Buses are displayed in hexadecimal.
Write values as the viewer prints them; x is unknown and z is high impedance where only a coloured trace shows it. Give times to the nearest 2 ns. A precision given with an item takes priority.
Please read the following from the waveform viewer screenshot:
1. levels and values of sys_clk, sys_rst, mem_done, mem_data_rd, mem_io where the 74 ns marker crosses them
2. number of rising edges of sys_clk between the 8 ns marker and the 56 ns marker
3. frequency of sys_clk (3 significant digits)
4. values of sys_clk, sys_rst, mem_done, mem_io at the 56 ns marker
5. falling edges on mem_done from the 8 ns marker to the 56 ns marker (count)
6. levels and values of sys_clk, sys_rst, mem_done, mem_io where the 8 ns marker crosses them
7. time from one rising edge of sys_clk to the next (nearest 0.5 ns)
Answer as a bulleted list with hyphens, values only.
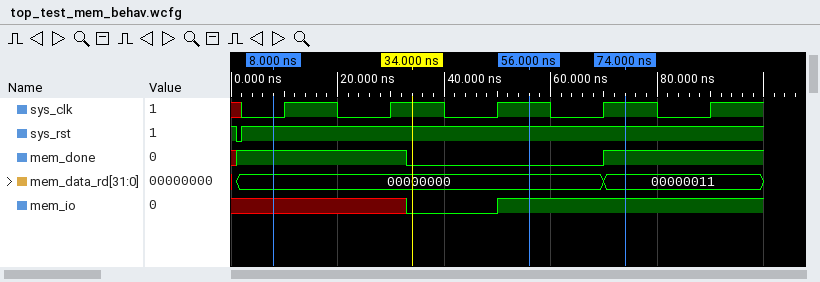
- sys_clk=1, sys_rst=1, mem_done=1, mem_data_rd=00000011, mem_io=1
- 3
- 50.0 MHz
- sys_clk=1, sys_rst=1, mem_done=0, mem_io=1
- 1
- sys_clk=0, sys_rst=1, mem_done=1, mem_io=x
- 20 ns
